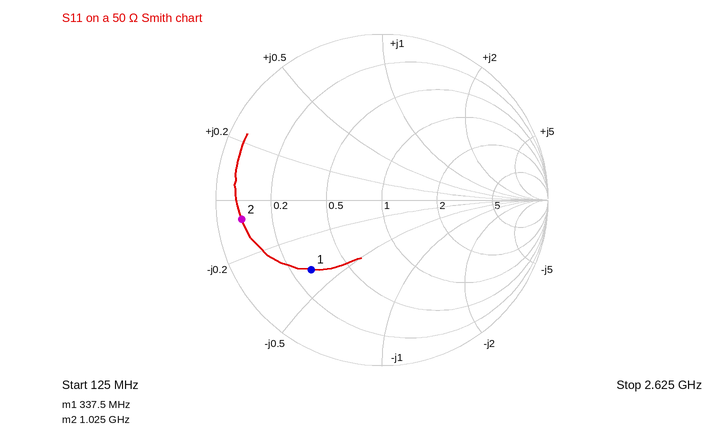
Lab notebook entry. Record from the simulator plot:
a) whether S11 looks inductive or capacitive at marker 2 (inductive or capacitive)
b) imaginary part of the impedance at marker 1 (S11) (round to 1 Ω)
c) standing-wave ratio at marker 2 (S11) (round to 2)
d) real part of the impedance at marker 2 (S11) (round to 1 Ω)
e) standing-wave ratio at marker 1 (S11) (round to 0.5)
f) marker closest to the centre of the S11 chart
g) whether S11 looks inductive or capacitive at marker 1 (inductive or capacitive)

capacitive
-19 Ω
12
4 Ω
4.0
marker 1
capacitive
